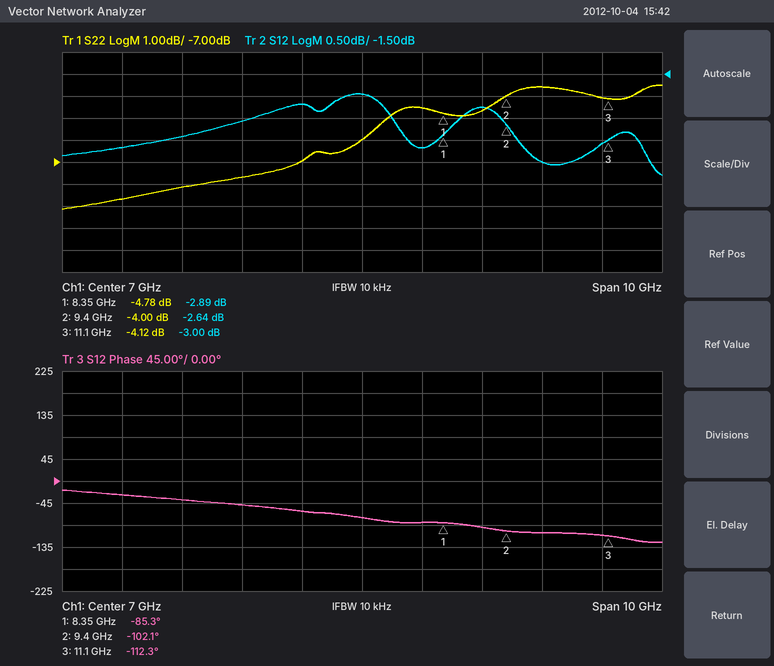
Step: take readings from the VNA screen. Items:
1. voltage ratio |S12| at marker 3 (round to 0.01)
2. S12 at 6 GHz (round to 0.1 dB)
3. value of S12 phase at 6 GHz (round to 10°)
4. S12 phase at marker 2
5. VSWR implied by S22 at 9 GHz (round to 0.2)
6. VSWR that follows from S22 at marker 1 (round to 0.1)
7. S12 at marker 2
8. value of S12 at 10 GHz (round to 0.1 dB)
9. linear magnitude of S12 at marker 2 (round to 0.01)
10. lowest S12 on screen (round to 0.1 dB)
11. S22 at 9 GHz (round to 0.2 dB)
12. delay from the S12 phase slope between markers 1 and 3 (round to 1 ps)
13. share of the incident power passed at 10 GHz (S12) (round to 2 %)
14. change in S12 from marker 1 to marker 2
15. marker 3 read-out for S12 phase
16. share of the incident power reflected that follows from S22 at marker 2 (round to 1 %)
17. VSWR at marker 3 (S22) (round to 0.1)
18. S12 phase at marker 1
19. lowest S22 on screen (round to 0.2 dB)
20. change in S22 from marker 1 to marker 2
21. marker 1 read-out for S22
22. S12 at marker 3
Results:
0.71
-2.2 dB
-60°
-102.1°
3.8
3.7
-2.64 dB
-3.5 dB
0.74
-3.8 dB
-4.6 dB
27 ps
44 %
0.25 dB
-112.3°
40 %
4.3
-85.3°
-9.2 dB
0.78 dB
-4.78 dB
-3.00 dB
